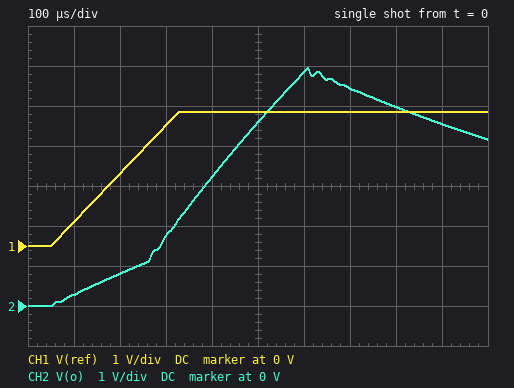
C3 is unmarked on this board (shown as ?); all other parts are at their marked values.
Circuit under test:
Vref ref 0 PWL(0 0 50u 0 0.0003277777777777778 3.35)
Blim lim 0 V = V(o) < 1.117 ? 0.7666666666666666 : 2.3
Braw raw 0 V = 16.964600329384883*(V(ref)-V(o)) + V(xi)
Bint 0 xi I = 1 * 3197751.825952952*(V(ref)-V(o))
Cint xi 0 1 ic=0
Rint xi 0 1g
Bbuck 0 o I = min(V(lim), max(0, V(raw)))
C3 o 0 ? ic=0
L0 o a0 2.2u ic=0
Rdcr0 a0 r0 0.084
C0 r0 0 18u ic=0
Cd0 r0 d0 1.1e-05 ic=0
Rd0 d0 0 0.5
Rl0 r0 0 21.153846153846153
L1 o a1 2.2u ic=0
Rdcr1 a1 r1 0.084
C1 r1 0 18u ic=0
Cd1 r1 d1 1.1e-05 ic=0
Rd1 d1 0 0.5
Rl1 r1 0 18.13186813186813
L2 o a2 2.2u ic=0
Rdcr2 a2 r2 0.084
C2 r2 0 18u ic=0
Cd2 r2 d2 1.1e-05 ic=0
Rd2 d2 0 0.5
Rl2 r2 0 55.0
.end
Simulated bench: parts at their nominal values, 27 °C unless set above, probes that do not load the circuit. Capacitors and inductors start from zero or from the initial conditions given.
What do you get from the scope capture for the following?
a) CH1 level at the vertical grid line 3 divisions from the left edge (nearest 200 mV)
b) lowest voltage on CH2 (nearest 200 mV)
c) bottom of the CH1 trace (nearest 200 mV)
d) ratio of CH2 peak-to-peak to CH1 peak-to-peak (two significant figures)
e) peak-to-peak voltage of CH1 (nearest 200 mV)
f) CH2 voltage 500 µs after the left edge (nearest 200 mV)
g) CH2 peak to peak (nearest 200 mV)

3.0 V
0 V
0 V
1.8
3.4 V
4.6 V
6.0 V
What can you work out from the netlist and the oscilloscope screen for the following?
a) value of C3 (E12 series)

47 µF
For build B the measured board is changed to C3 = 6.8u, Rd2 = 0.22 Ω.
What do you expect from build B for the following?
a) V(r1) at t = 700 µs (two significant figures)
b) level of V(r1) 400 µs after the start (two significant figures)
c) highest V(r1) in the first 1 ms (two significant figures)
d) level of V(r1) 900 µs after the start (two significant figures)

3.5 V
4.8 V
5.1 V
2.7 V
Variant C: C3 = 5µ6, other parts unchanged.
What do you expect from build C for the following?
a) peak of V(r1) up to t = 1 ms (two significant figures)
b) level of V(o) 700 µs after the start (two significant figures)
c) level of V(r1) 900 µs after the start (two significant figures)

5.1 V
3.5 V
2.7 V
